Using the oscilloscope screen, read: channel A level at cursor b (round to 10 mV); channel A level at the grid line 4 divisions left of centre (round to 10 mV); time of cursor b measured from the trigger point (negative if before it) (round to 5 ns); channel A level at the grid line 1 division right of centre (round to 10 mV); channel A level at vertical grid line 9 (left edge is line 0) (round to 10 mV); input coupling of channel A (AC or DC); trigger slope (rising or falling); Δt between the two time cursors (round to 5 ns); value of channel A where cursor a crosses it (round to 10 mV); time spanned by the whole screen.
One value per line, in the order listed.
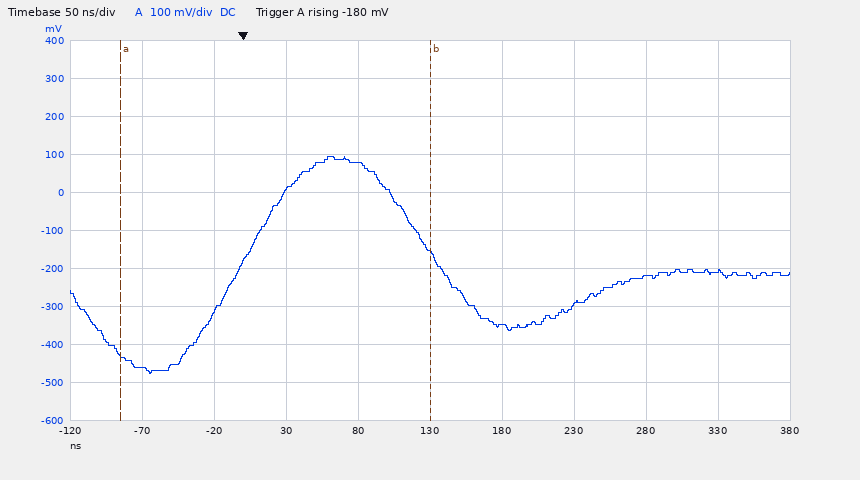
-160 mV
-460 mV
+130 ns
-350 mV
-210 mV
DC
rising
215 ns
-430 mV
500 ns
